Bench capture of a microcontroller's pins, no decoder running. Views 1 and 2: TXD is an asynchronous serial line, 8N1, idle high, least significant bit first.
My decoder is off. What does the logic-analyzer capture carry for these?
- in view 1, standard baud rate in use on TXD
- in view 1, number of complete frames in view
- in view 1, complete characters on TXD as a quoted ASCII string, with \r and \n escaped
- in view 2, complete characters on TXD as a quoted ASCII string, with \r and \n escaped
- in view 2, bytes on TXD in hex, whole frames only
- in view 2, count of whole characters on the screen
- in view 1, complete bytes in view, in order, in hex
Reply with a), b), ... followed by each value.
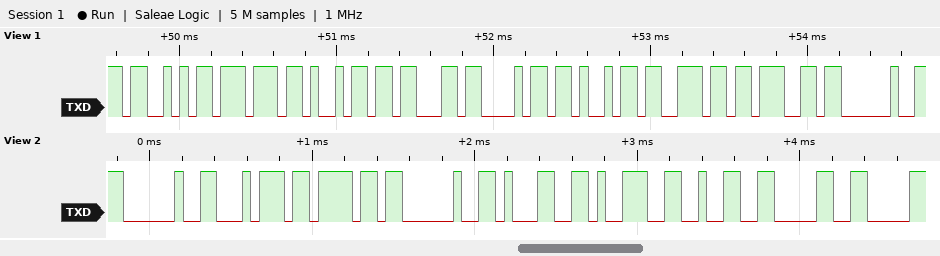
a) 19200 baud
b) 9
c) "Swiching "
d) " to 1920"
e) 0x20 0x74 0x6F 0x20 0x31 0x39 0x32 0x30
f) 8
g) 0x53 0x77 0x69 0x63 0x68 0x69 0x6E 0x67 0x20
